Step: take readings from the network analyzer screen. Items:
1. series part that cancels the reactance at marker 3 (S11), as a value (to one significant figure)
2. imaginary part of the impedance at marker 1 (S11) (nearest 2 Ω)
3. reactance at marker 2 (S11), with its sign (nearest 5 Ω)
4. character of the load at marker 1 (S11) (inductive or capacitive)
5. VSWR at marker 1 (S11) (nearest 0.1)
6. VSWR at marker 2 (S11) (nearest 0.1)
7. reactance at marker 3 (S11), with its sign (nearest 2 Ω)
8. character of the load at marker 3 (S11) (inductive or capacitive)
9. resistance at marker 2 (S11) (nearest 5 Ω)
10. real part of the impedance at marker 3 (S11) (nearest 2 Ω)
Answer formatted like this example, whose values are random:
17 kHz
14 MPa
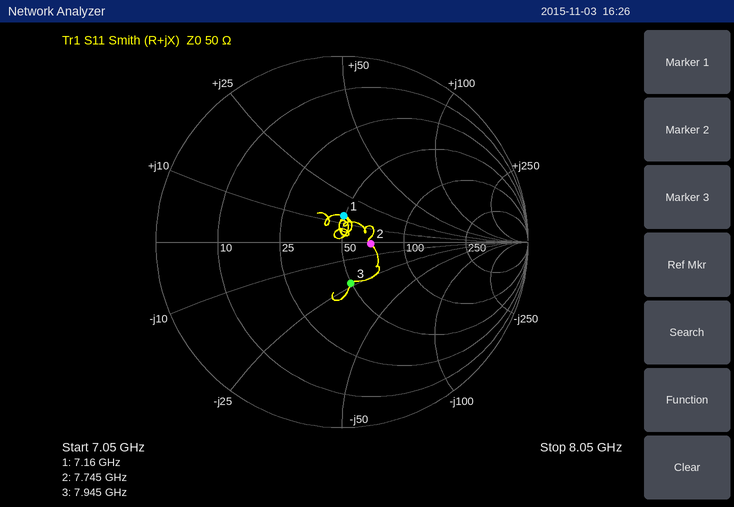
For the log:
500 pH
+14 Ω
0 Ω
inductive
1.3
1.4
-24 Ω
capacitive
70 Ω
50 Ω
